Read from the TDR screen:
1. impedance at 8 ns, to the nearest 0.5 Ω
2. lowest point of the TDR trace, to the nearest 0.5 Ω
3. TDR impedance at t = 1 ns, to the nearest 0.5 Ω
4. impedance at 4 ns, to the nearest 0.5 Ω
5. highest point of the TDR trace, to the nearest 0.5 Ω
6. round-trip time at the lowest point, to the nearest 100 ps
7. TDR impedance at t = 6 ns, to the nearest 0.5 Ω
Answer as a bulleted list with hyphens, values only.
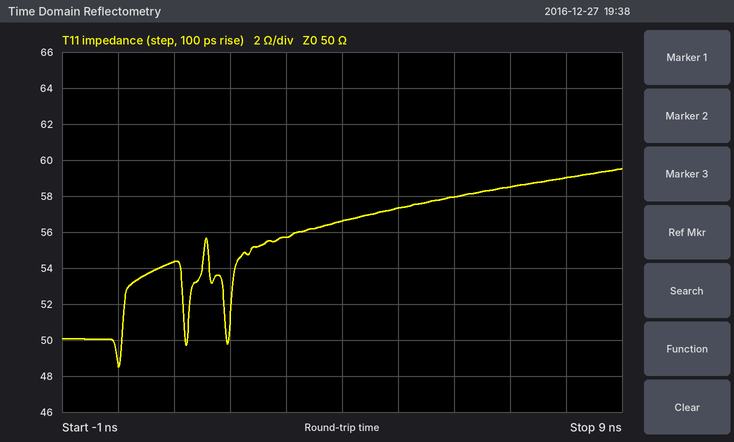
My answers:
- 59.0 Ω
- 48.5 Ω
- 54.5 Ω
- 56.5 Ω
- 59.5 Ω
- 0.0 ns
- 58.0 Ω
